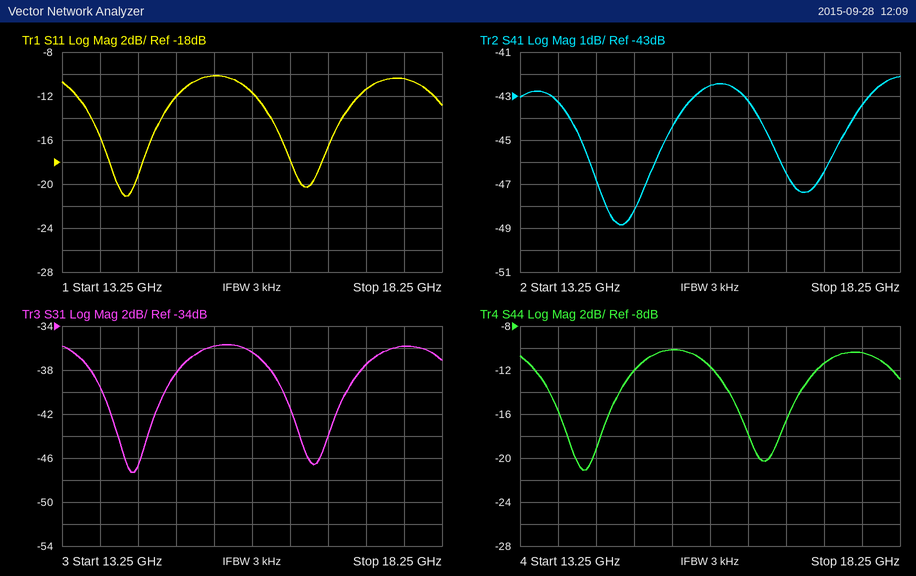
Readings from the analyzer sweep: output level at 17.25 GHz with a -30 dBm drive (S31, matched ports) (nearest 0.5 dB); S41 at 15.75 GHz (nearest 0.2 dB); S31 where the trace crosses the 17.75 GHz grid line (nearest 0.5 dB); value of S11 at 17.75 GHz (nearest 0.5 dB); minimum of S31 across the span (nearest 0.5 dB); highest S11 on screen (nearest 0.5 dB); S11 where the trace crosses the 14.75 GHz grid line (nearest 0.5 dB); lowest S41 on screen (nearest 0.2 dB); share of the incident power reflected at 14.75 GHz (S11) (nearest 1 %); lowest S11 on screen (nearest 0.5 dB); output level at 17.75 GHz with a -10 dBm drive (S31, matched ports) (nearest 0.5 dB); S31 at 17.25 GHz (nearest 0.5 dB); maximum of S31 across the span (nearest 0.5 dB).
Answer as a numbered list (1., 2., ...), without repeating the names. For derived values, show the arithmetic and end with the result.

1. -30 dBm + (-37.5 dB) = -67.5 dBm
2. -42.6 dB
3. -36.0 dB
4. -10.5 dB
5. -47.5 dB
6. -10.0 dB
7. -12.0 dB
8. -48.8 dB
9. 10^(-12/10) ≈ 6 %
10. -21.0 dB
11. -10 dBm + (-36.0 dB) = -46.0 dBm
12. -37.5 dB
13. -35.5 dB
